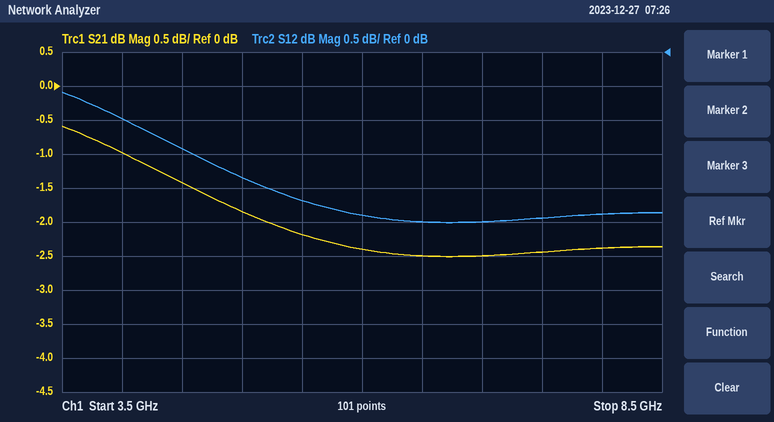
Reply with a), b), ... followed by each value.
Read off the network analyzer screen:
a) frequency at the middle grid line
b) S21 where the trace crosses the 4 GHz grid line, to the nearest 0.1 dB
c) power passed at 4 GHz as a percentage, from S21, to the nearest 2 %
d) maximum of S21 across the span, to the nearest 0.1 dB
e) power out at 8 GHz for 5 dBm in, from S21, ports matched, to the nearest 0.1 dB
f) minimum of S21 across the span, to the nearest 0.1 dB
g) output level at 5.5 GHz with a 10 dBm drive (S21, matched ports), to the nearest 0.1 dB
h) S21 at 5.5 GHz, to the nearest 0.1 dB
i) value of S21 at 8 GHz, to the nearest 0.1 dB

a) 6 GHz
b) -1.0 dB
c) 80 %
d) -0.6 dB
e) 2.6 dBm
f) -2.5 dB
g) 7.8 dBm
h) -2.2 dB
i) -2.4 dB
